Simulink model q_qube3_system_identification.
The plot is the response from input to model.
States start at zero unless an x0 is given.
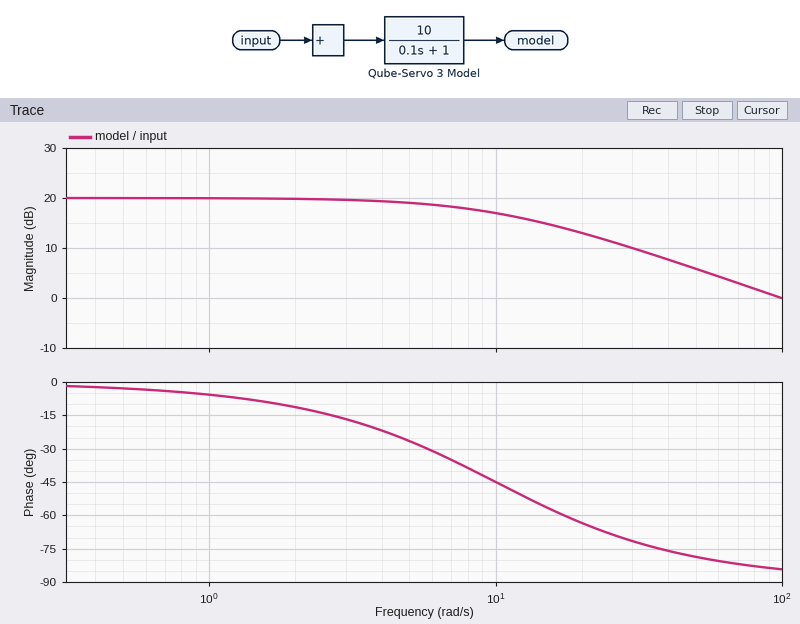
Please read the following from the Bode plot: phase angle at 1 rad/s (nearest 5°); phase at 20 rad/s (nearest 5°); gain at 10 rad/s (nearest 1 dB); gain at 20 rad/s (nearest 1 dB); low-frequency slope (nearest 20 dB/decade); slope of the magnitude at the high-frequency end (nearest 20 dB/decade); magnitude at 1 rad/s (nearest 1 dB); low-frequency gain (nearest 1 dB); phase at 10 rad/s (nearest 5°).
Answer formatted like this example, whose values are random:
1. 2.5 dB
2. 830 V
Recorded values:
1. -5°
2. -65°
3. 17 dB
4. 13 dB
5. 0 dB/decade
6. -20 dB/decade
7. 20 dB
8. 20 dB
9. -45°
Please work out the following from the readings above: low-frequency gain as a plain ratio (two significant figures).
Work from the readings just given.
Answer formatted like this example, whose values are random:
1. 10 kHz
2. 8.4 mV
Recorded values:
1. 10
